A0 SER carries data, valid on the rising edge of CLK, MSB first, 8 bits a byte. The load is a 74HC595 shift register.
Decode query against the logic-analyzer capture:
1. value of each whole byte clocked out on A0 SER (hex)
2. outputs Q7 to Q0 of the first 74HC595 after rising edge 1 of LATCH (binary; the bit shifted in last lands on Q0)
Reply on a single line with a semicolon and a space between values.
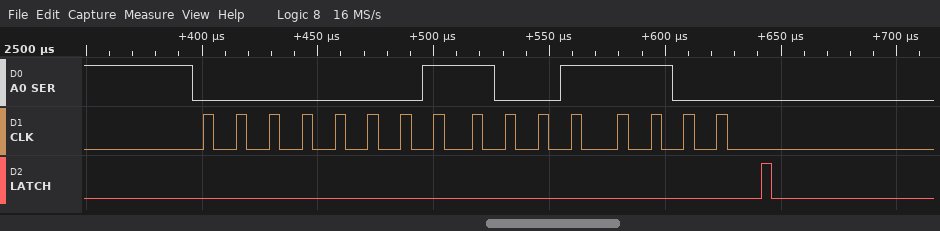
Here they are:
01 9C; 10011100
